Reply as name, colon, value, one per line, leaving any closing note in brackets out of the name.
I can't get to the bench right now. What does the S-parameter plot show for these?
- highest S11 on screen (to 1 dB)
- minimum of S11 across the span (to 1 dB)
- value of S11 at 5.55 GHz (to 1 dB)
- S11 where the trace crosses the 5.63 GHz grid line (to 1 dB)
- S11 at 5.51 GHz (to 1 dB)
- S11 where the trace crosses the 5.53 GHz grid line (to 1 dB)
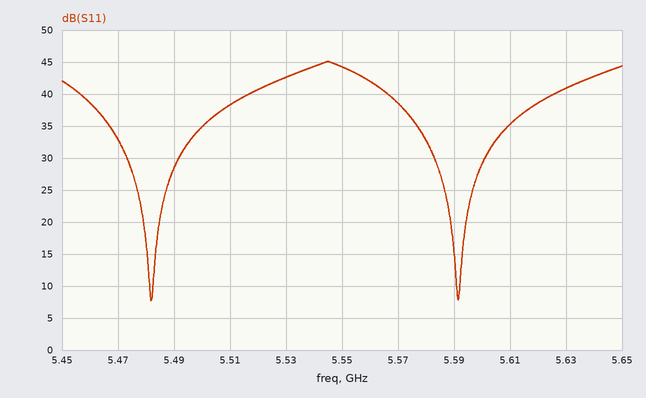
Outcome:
highest S11 on screen: 45 dB
minimum of S11 across the span: 8 dB
value of S11 at 5.55 GHz: 44 dB
S11 where the trace crosses the 5.63 GHz grid line: 41 dB
S11 at 5.51 GHz: 38 dB
S11 where the trace crosses the 5.53 GHz grid line: 43 dB
